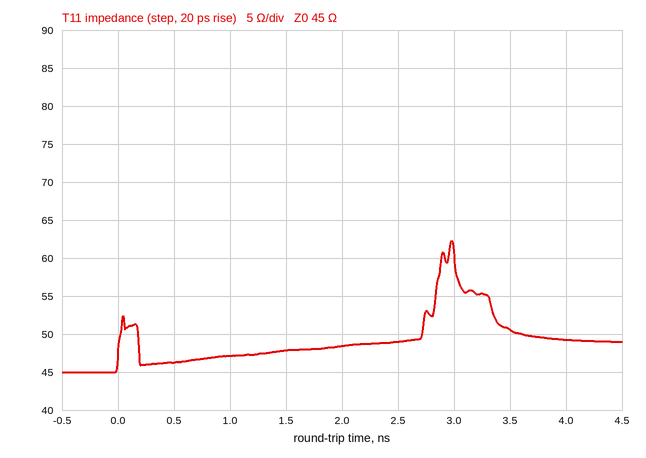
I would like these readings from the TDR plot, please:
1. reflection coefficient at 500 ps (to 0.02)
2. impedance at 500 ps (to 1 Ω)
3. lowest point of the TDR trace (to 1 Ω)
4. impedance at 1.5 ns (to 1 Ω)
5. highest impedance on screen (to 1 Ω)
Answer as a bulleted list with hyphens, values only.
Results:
- +0.02
- 46 Ω
- 45 Ω
- 48 Ω
- 62 Ω
